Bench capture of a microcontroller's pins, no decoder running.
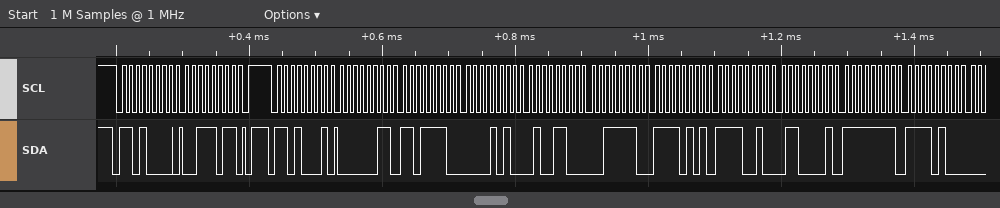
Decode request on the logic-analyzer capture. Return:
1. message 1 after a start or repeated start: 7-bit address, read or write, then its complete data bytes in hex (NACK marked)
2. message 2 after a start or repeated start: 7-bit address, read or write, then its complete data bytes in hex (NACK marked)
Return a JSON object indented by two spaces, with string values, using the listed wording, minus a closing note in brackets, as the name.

{
  "message 1 after a start or repeated start: 7-bit address, read or write, then its complete data bytes in hex": "0x68 write: 3B",
  "message 2 after a start or repeated start: 7-bit address, read or write, then its complete data bytes in hex": "0x68 read: 03 DE 0A 4C 3E F5 F2 61 FF F4"
}
